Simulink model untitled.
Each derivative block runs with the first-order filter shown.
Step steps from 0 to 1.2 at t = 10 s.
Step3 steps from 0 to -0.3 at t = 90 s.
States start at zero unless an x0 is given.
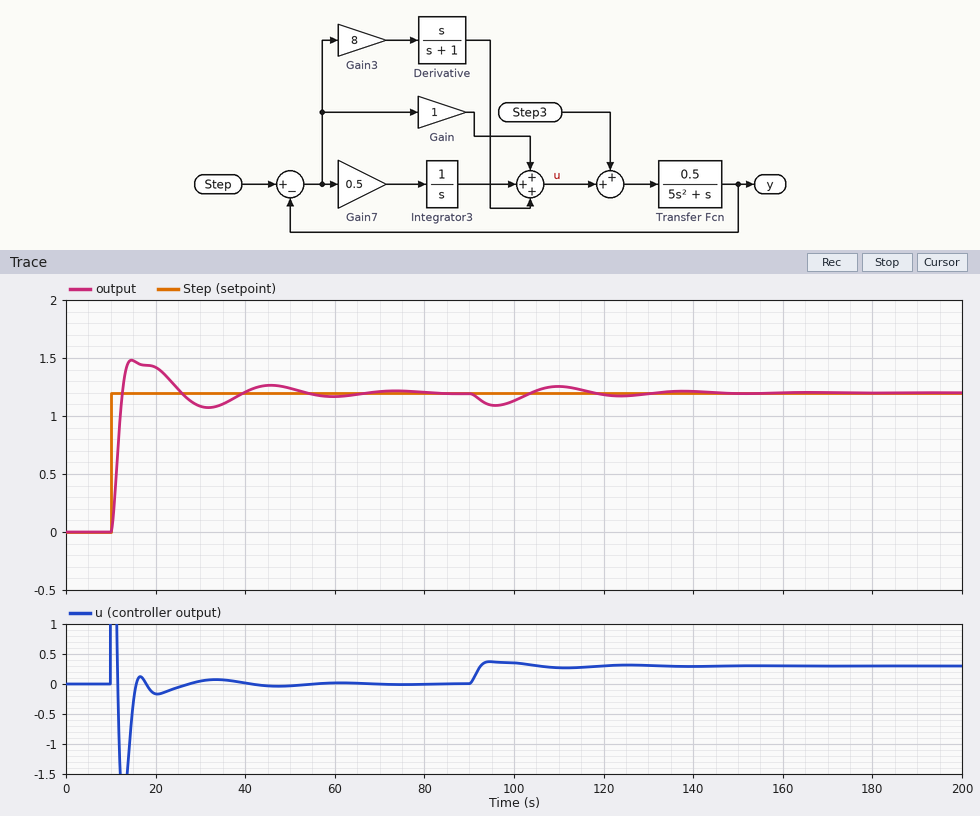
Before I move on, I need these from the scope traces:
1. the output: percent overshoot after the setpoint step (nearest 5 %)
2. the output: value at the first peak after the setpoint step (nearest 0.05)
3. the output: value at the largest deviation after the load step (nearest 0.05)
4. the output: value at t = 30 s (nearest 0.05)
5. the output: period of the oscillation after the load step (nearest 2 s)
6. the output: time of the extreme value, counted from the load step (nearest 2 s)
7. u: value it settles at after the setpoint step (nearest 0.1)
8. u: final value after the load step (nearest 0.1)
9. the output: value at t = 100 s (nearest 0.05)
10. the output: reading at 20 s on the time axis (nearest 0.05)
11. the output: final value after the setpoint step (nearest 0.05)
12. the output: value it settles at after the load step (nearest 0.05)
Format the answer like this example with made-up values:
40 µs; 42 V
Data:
25 %; 1.50; 1.10; 1.10; 28 s; 6 s; 0.0; 0.3; 1.15; 1.40; 1.20; 1.20
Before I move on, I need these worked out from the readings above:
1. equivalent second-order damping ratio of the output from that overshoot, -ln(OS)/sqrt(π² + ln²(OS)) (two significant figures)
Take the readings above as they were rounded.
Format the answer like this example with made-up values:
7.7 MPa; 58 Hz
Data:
0.40
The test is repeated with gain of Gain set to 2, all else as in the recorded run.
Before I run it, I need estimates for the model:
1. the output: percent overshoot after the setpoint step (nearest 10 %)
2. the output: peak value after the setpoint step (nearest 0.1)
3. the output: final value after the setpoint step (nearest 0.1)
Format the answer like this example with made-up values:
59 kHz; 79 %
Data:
30 %; 1.6; 1.2
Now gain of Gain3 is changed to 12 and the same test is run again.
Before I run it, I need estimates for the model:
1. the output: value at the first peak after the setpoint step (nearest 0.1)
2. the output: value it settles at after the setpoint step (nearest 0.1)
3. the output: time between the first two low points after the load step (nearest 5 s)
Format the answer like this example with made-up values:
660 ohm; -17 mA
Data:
1.4; 1.2; 35 s
